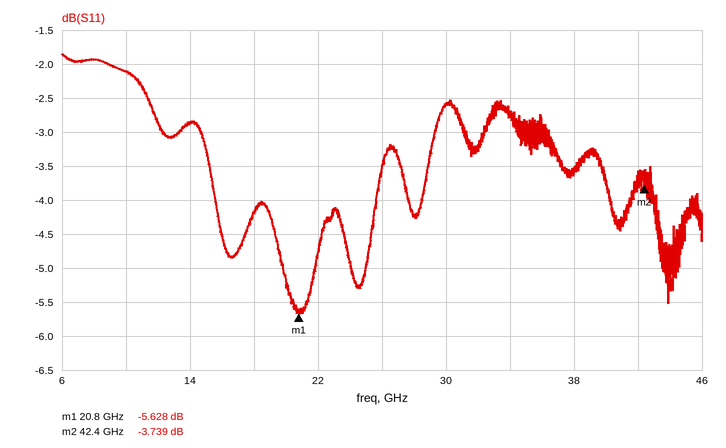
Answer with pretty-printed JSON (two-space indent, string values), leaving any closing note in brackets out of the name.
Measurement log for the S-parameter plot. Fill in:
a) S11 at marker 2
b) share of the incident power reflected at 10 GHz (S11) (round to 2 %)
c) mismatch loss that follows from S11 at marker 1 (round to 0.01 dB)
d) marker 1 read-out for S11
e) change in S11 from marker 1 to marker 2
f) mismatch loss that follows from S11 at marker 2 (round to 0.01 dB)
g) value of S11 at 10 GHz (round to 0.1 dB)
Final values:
{
  "S11 at marker 2": "-3.739 dB",
  "share of the incident power reflected at 10 GHz (S11)": "62 %",
  "mismatch loss that follows from S11 at marker 1": "1.39 dB",
  "marker 1 read-out for S11": "-5.628 dB",
  "change in S11 from marker 1 to marker 2": "1.889 dB",
  "mismatch loss that follows from S11 at marker 2": "2.39 dB",
  "value of S11 at 10 GHz": "-2.1 dB"
}
